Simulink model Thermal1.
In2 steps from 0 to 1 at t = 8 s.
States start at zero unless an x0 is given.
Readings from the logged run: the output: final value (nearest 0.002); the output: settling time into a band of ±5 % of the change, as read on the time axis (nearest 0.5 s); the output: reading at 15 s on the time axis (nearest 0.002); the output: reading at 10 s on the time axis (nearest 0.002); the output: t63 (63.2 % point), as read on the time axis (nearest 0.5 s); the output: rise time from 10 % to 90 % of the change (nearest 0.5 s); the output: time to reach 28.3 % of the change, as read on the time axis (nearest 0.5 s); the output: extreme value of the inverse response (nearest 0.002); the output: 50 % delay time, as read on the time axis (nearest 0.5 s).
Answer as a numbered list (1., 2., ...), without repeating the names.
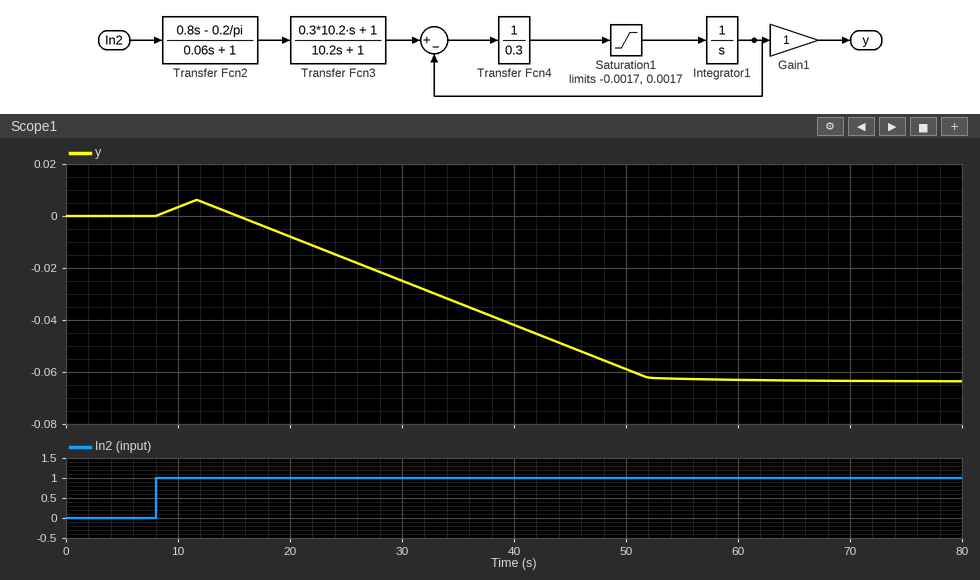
1. -0.064
2. 51.0 s
3. 0.000
4. 0.004
5. 39.0 s
6. 30.0 s
7. 26.0 s
8. 0.006
9. 34.0 s
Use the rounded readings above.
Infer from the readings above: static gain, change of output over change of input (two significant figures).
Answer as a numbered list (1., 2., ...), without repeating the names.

1. -0.064
